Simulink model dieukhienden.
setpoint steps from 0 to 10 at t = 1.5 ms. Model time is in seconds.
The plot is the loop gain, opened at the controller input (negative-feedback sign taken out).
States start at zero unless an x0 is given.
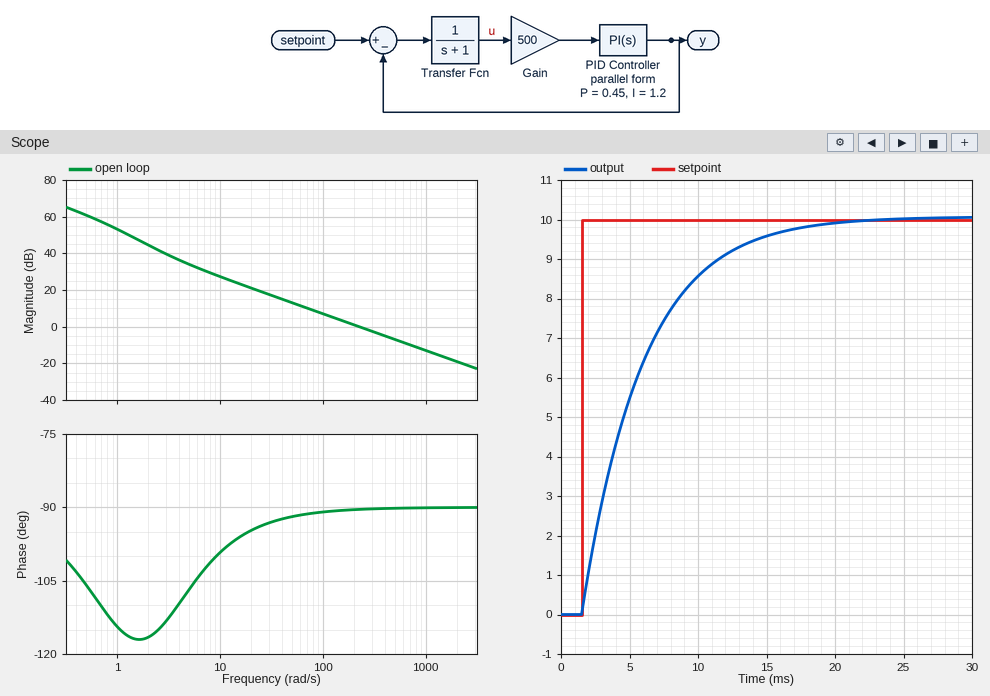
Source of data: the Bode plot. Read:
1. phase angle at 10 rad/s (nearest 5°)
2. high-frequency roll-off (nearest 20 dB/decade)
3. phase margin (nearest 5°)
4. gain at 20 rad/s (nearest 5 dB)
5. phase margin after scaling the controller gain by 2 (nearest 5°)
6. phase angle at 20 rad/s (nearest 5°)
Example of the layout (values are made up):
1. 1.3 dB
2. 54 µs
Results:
1. -100°
2. -20 dB/decade
3. 90°
4. 20 dB
5. 90°
6. -95°
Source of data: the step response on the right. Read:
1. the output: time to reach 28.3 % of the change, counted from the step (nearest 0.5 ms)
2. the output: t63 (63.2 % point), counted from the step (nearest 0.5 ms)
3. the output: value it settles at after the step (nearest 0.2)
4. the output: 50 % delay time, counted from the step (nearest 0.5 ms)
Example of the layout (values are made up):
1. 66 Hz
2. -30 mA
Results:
1. 1.5 ms
2. 4.5 ms
3. 10.0
4. 3.0 ms
